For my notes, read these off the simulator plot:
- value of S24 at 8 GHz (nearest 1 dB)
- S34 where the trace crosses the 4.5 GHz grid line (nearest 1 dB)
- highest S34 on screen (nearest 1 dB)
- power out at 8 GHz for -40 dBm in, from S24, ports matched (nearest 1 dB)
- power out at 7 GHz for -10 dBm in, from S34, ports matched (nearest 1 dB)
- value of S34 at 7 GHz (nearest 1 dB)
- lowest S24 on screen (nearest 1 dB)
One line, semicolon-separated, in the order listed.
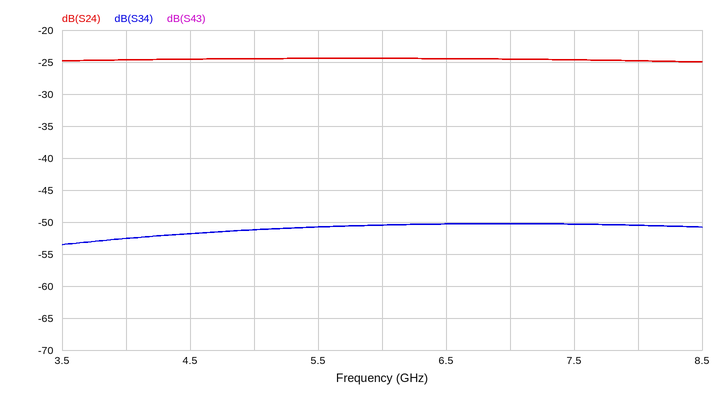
-25 dB; -52 dB; -50 dB; -65 dBm; -60 dBm; -50 dB; -25 dB
